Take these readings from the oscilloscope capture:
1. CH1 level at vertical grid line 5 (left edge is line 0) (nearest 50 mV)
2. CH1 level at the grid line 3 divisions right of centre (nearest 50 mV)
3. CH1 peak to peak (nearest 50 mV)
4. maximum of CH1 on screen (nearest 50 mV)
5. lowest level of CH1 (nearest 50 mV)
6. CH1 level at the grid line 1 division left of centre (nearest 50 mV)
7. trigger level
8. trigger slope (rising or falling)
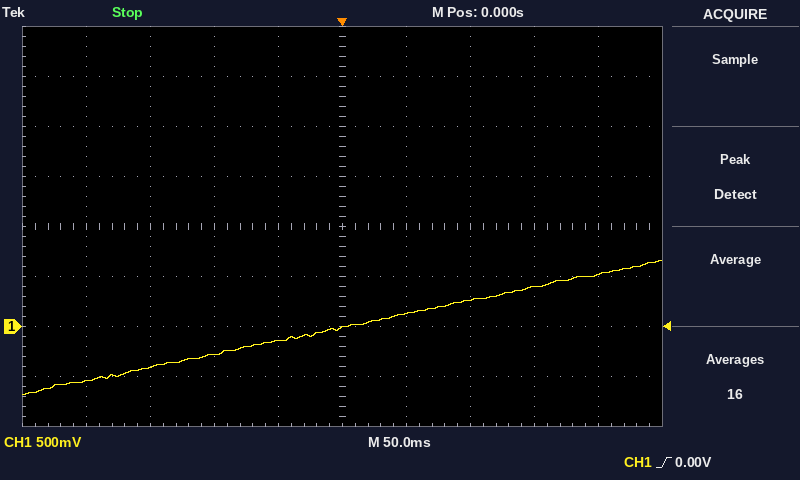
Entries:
0 mV
400 mV
1.35 V
650 mV
-700 mV
-150 mV
0.00 V
rising
